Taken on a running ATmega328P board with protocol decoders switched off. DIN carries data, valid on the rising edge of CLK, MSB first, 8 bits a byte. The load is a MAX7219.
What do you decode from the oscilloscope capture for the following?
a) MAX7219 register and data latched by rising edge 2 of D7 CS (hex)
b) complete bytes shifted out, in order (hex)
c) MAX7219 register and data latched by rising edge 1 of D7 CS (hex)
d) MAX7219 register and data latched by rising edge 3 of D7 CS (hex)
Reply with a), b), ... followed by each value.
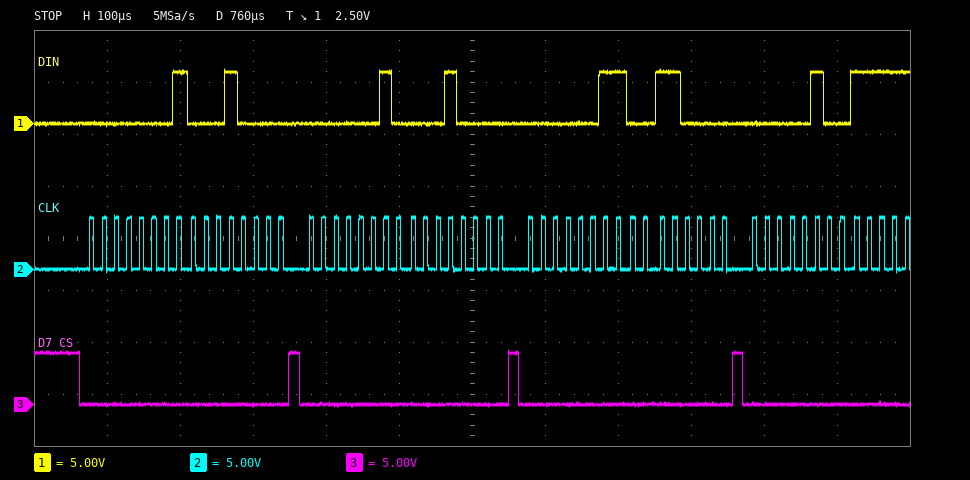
a) register 0x2, data 0x10
b) 01 10 02 10 03 30 04
c) register 0x1, data 0x10
d) register 0x3, data 0x30
